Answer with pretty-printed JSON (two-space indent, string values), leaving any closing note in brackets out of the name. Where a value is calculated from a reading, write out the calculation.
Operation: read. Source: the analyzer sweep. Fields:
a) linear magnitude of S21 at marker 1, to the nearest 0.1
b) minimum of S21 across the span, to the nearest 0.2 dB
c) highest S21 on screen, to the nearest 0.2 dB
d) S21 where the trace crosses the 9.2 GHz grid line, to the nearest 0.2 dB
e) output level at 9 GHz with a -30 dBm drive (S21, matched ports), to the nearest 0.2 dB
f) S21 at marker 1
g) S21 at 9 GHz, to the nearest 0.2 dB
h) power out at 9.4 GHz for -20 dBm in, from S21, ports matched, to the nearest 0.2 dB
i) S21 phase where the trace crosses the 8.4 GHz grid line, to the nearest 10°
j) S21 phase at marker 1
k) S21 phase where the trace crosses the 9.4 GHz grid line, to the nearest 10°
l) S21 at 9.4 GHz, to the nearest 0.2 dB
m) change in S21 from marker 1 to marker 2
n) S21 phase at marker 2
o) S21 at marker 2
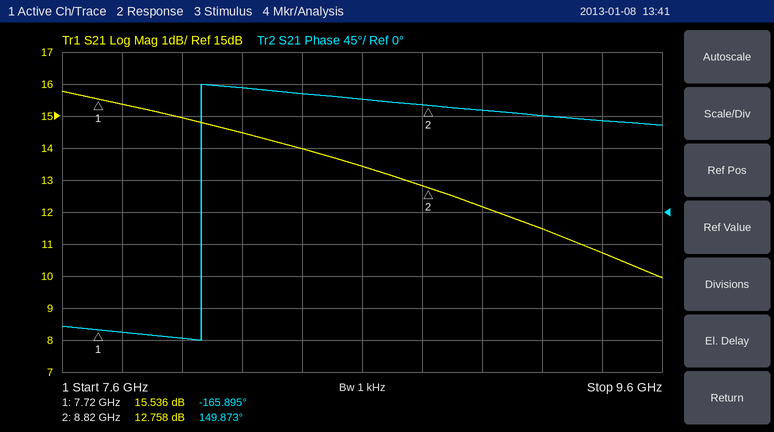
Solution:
{
  "linear magnitude of S21 at marker 1, to the nearest 0.1": "10^(15.536/20) ≈ 6.0",
  "minimum of S21 across the span, to the nearest 0.2 dB": "10.0 dB",
  "highest S21 on screen, to the nearest 0.2 dB": "15.8 dB",
  "S21 where the trace crosses the 9.2 GHz grid line, to the nearest 0.2 dB": "11.4 dB",
  "output level at 9 GHz with a -30 dBm drive (S21, matched ports), to the nearest 0.2 dB": "-30 dBm + (12.2 dB) = -17.8 dBm",
  "S21 at marker 1": "15.536 dB",
  "S21 at 9 GHz, to the nearest 0.2 dB": "12.2 dB",
  "power out at 9.4 GHz for -20 dBm in, from S21, ports matched, to the nearest 0.2 dB": "-20 dBm + (10.8 dB) = -9.2 dBm",
  "S21 phase where the trace crosses the 8.4 GHz grid line, to the nearest 10°": "170°",
  "S21 phase at marker 1": "-165.895°",
  "S21 phase where the trace crosses the 9.4 GHz grid line, to the nearest 10°": "130°",
  "S21 at 9.4 GHz, to the nearest 0.2 dB": "10.8 dB",
  "change in S21 from marker 1 to marker 2": "12.758 − (15.536) = -2.778 dB",
  "S21 phase at marker 2": "149.873°",
  "S21 at marker 2": "12.758 dB"
}
